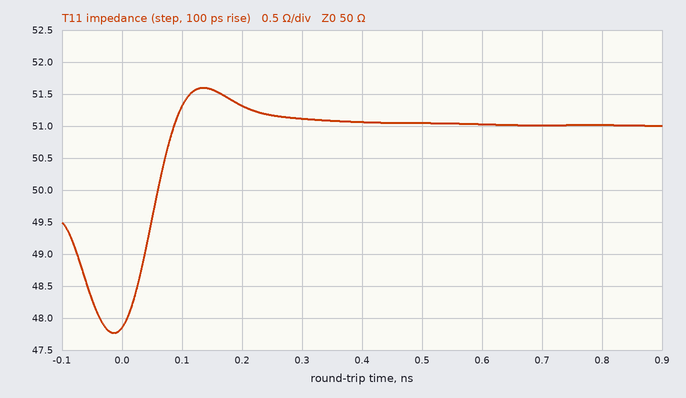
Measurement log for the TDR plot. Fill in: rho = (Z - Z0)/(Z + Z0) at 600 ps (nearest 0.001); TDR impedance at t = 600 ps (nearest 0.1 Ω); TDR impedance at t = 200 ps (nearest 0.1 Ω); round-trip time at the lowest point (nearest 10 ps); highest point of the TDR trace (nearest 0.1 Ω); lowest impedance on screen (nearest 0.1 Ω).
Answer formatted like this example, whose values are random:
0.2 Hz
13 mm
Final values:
+0.010
51.0 Ω
51.3 Ω
-10 ps
51.6 Ω
47.8 Ω
